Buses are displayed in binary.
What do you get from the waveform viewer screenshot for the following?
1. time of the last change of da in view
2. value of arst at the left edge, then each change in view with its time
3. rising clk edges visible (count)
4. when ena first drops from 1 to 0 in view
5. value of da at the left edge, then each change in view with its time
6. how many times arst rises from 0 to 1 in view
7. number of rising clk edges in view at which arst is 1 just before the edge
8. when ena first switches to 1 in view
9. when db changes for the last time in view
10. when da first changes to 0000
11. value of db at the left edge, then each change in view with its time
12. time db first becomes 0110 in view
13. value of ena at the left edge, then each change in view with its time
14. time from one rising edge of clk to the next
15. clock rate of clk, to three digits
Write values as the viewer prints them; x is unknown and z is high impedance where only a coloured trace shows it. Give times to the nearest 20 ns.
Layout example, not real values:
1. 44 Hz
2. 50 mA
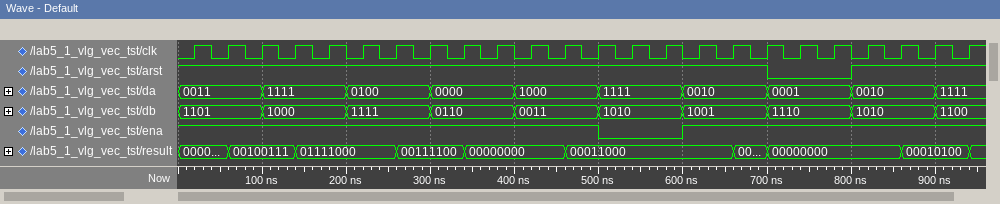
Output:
1. 900 ns
2. 1, 0 at 700 ns, 1 at 800 ns
3. 24
4. 500 ns
5. 0011, 1111 at 100 ns, 0100 at 200 ns, 0000 at 300 ns, 1000 at 400 ns, 1111 at 500 ns, 0010 at 600 ns, 0001 at 700 ns, 0010 at 800 ns, 1111 at 900 ns
6. 1
7. 22
8. 600 ns
9. 900 ns
10. 300 ns
11. 1101, 1000 at 100 ns, 1111 at 200 ns, 0110 at 300 ns, 0011 at 400 ns, 1010 at 500 ns, 1001 at 600 ns, 1110 at 700 ns, 1010 at 800 ns, 1100 at 900 ns
12. 300 ns
13. 1, 0 at 500 ns, 1 at 600 ns
14. 40 ns
15. 25.0 MHz
